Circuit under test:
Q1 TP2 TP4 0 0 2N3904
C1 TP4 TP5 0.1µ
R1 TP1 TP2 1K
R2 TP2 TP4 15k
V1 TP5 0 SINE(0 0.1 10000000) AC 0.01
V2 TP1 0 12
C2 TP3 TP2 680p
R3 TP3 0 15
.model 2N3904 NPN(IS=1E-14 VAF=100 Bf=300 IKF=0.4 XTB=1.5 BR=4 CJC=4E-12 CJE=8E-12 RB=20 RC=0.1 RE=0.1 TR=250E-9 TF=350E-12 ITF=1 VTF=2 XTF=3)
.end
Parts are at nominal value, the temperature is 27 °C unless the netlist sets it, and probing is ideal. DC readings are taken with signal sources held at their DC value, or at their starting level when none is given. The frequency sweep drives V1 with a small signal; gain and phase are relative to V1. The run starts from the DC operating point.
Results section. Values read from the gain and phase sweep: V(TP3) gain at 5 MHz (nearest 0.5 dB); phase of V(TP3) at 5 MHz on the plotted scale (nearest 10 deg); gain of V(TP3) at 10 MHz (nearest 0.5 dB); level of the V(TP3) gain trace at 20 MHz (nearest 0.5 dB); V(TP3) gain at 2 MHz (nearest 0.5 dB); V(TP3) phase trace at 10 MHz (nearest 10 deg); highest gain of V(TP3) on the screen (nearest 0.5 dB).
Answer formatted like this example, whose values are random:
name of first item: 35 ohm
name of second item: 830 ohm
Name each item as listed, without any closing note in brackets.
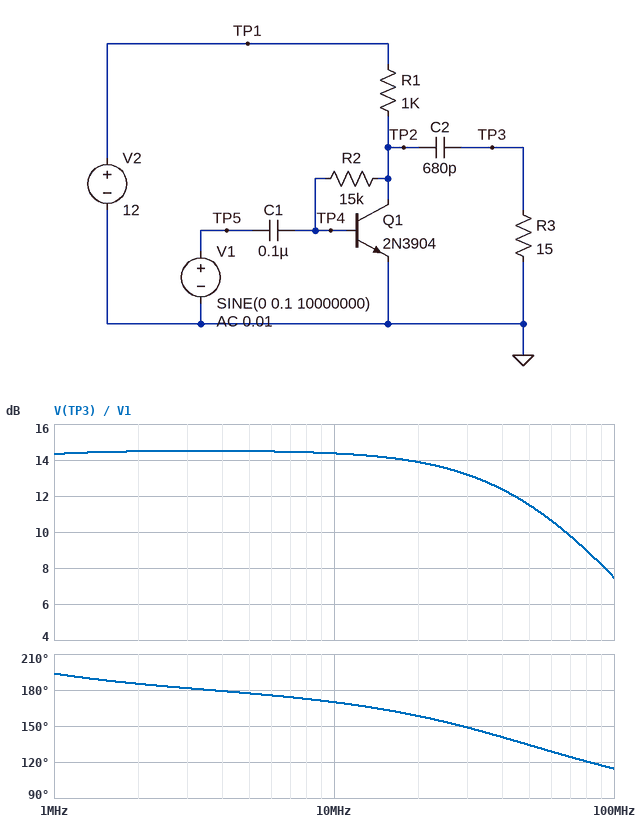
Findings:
V(TP3) gain at 5 MHz: 14.5 dB
phase of V(TP3) at 5 MHz on the plotted scale: 180 deg
gain of V(TP3) at 10 MHz: 14.5 dB
level of the V(TP3) gain trace at 20 MHz: 14.0 dB
V(TP3) gain at 2 MHz: 14.5 dB
V(TP3) phase trace at 10 MHz: 170 deg
highest gain of V(TP3) on the screen: 14.5 dB
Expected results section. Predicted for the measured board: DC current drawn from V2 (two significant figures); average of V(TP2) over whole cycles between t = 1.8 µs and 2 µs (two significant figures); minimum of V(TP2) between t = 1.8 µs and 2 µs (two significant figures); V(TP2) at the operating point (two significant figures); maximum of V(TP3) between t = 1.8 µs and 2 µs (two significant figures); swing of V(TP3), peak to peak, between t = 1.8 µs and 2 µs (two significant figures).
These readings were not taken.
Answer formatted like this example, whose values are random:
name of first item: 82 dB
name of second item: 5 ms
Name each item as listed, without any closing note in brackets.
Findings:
DC current drawn from V2: 11 mA
average of V(TP2) over whole cycles between t = 1.8 µs and 2 µs: 180 mV
minimum of V(TP2) between t = 1.8 µs and 2 µs: 88 mV
V(TP2) at the operating point: 1.3 V
maximum of V(TP3) between t = 1.8 µs and 2 µs: 170 mV
swing of V(TP3), peak to peak, between t = 1.8 µs and 2 µs: 290 mV
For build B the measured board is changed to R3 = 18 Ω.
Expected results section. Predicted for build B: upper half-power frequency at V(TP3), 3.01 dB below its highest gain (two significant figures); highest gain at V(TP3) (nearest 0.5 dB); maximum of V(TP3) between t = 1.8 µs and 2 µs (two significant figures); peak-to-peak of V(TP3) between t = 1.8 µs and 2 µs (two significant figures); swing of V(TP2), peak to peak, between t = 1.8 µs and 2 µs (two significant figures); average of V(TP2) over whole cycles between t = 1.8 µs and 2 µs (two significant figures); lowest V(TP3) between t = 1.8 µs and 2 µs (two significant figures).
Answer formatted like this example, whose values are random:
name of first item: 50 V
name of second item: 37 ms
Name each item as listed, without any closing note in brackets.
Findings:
upper half-power frequency at V(TP3), 3.01 dB below its highest gain: 49 MHz
highest gain at V(TP3): 16.0 dB
maximum of V(TP3) between t = 1.8 µs and 2 µs: 200 mV
peak-to-peak of V(TP3) between t = 1.8 µs and 2 µs: 330 mV
swing of V(TP2), peak to peak, between t = 1.8 µs and 2 µs: 380 mV
average of V(TP2) over whole cycles between t = 1.8 µs and 2 µs: 190 mV
lowest V(TP3) between t = 1.8 µs and 2 µs: -130 mV
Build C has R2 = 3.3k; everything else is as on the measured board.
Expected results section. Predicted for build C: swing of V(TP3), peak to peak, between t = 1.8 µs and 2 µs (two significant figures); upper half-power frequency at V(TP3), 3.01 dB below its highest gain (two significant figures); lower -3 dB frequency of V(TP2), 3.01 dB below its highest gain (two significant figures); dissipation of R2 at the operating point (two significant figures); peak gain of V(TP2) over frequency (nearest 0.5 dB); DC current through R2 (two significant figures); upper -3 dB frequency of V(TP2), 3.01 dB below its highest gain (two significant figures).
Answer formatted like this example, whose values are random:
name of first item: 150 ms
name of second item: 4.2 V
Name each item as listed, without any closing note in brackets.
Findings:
swing of V(TP3), peak to peak, between t = 1.8 µs and 2 µs: 310 mV
upper half-power frequency at V(TP3), 3.01 dB below its highest gain: 48 MHz
lower -3 dB frequency of V(TP2), 3.01 dB below its highest gain: 100 kHz
dissipation of R2 at the operating point: 4.8 µW
peak gain of V(TP2) over frequency: 48.5 dB
DC current through R2: 38 µA
upper -3 dB frequency of V(TP2), 3.01 dB below its highest gain: 420 kHz
